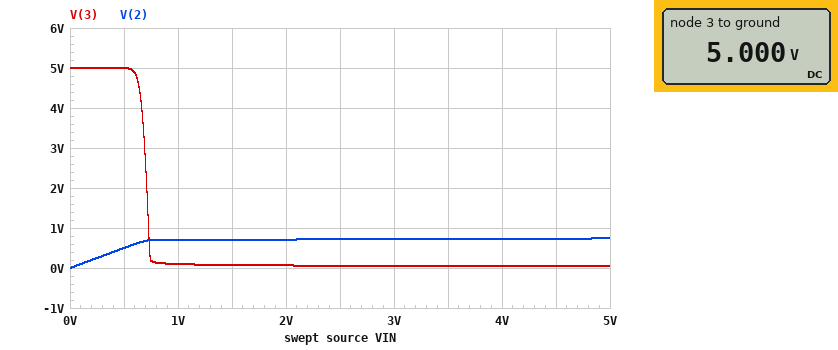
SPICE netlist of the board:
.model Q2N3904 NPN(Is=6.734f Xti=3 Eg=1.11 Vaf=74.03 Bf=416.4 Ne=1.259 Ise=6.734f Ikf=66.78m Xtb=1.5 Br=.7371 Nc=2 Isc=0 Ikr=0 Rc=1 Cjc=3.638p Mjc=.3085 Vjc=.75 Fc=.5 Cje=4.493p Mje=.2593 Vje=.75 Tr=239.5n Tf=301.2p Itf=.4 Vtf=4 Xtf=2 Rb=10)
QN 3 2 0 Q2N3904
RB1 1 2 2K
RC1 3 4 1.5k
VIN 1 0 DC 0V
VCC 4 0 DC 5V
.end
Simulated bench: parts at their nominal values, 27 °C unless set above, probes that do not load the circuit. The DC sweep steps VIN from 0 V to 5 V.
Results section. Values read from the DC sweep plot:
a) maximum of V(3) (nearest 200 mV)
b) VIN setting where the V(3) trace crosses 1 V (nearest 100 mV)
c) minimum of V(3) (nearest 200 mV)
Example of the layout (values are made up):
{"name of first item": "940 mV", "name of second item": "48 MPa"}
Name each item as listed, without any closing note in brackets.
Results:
{"maximum of V(3)": "5.0 V", "VIN setting where the V(3) trace crosses 1 V": "700 mV", "minimum of V(3)": "0 V"}
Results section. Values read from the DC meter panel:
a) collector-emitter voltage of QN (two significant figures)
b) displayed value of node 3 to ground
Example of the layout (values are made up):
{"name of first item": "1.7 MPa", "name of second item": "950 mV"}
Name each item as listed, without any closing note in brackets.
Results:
{"collector-emitter voltage of QN": "5.0 V", "displayed value of node 3 to ground": "5.000 V"}
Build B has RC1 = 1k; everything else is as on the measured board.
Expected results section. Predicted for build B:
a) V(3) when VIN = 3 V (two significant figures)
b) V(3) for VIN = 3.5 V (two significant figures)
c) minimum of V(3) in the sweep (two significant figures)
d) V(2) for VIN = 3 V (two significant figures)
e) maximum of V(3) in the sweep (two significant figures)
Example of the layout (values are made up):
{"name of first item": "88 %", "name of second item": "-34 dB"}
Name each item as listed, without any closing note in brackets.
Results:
{"V(3) when VIN = 3 V": "63 mV", "V(3) for VIN = 3.5 V": "59 mV", "minimum of V(3) in the sweep": "52 mV", "V(2) for VIN = 3 V": "730 mV", "maximum of V(3) in the sweep": "5.0 V"}
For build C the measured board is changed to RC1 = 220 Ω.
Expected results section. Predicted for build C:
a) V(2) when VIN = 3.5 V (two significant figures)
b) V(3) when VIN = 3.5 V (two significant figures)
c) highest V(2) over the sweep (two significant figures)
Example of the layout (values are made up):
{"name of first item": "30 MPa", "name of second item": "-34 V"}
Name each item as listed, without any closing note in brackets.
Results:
{"V(2) when VIN = 3.5 V": "770 mV", "V(3) when VIN = 3.5 V": "120 mV", "highest V(2) over the sweep": "780 mV"}
